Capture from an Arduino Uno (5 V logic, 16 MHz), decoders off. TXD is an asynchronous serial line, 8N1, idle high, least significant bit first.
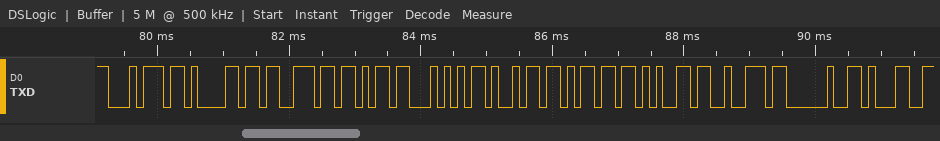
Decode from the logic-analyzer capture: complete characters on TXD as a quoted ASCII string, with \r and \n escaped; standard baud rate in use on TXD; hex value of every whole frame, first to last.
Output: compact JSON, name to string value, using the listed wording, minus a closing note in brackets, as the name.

{"complete characters on TXD as a quoted ASCII string, with \\r and \\n escaped": "\"taskTimer 1\"", "standard baud rate in use on TXD": "9600 baud", "hex value of every whole frame, first to last": "74 61 73 6B 54 69 6D 65 72 20 31"}
